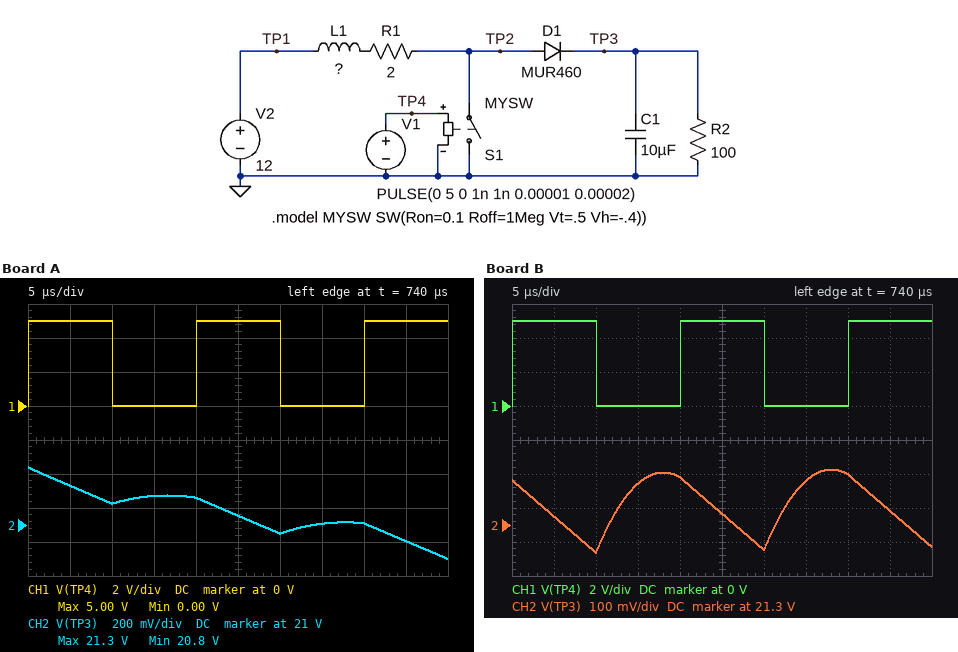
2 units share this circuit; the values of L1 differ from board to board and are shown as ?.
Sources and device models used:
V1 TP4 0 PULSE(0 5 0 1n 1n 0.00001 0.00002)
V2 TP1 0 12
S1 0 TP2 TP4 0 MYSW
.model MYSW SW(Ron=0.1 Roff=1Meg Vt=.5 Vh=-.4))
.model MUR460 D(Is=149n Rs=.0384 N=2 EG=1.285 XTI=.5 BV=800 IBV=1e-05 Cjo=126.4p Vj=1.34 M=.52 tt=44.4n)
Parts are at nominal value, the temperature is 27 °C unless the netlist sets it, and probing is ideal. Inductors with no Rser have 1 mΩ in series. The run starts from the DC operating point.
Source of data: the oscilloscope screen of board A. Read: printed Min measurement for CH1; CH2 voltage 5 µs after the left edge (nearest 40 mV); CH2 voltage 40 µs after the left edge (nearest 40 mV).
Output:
0.00 V
21.24 V
21.00 V
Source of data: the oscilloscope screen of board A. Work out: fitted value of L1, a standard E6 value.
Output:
470 µH
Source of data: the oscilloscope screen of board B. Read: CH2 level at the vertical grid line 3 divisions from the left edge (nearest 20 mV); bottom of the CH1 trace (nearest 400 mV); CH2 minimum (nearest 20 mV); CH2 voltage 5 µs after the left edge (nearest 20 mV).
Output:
21.42 V
0 V
21.22 V
21.32 V
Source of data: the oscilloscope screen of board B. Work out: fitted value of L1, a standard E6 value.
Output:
150 µH
